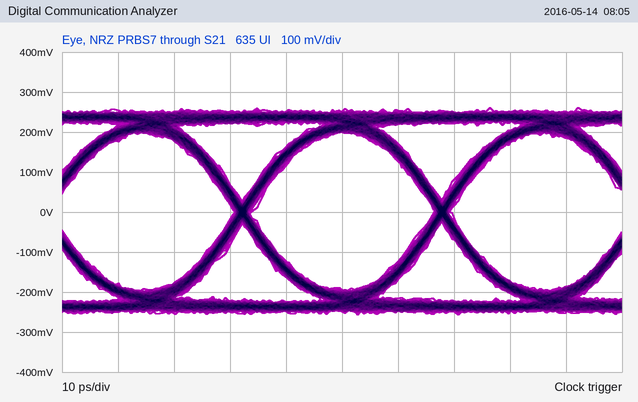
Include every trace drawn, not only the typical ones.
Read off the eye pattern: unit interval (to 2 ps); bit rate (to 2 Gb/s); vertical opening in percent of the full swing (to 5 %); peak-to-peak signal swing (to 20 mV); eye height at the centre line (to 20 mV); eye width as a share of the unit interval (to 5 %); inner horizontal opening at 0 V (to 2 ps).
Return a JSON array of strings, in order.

["36 ps", "28 Gb/s", "75 %", "520 mV", "400 mV", "90 %", "32 ps"]
